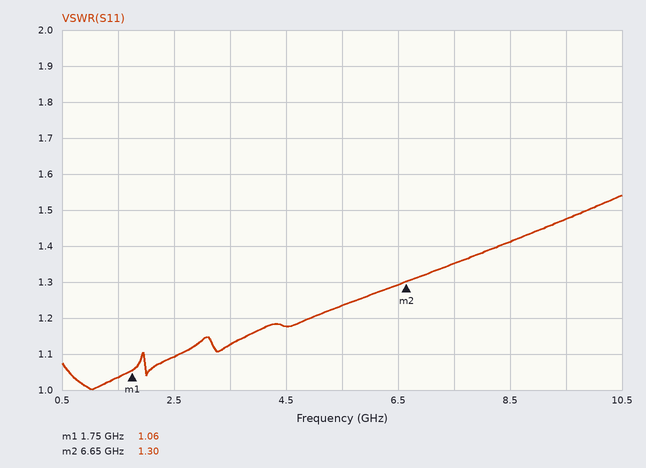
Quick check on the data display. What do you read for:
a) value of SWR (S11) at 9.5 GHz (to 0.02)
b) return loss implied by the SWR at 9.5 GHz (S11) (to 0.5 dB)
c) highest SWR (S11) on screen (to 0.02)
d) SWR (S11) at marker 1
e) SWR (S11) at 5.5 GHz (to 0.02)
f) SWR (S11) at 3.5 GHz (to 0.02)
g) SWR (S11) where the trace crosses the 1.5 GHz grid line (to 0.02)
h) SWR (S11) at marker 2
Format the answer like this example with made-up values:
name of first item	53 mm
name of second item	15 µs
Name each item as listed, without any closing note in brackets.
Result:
value of SWR (S11) at 9.5 GHz	1.48
return loss implied by the SWR at 9.5 GHz (S11)	14.5 dB
highest SWR (S11) on screen	1.54
SWR (S11) at marker 1	1.06
SWR (S11) at 5.5 GHz	1.24
SWR (S11) at 3.5 GHz	1.12
SWR (S11) where the trace crosses the 1.5 GHz grid line	1.04
SWR (S11) at marker 2	1.30
